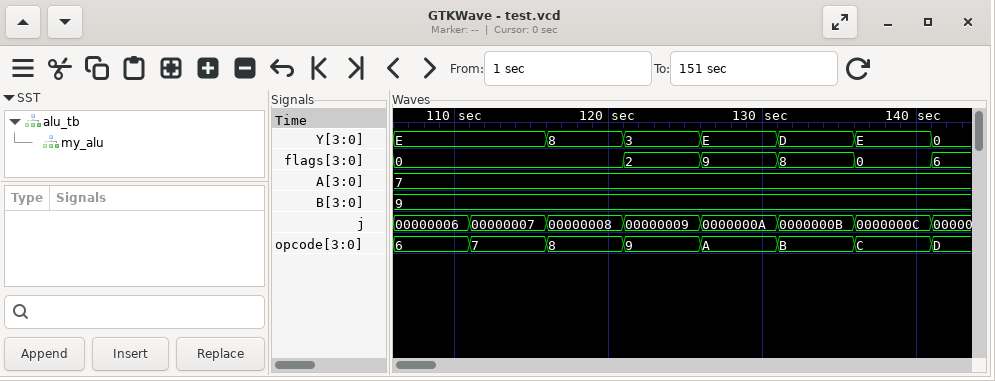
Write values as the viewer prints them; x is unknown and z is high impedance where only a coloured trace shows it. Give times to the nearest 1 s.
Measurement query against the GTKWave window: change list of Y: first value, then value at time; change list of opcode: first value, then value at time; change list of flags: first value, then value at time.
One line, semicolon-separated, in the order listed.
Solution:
E, 8 at 116 s, 3 at 121 s, E at 126 s, D at 131 s, E at 136 s, 0 at 141 s; 6, 7 at 111 s, 8 at 116 s, 9 at 121 s, A at 126 s, B at 131 s, C at 136 s, D at 141 s; 0, 2 at 121 s, 9 at 126 s, 8 at 131 s, 0 at 136 s, 6 at 141 s
